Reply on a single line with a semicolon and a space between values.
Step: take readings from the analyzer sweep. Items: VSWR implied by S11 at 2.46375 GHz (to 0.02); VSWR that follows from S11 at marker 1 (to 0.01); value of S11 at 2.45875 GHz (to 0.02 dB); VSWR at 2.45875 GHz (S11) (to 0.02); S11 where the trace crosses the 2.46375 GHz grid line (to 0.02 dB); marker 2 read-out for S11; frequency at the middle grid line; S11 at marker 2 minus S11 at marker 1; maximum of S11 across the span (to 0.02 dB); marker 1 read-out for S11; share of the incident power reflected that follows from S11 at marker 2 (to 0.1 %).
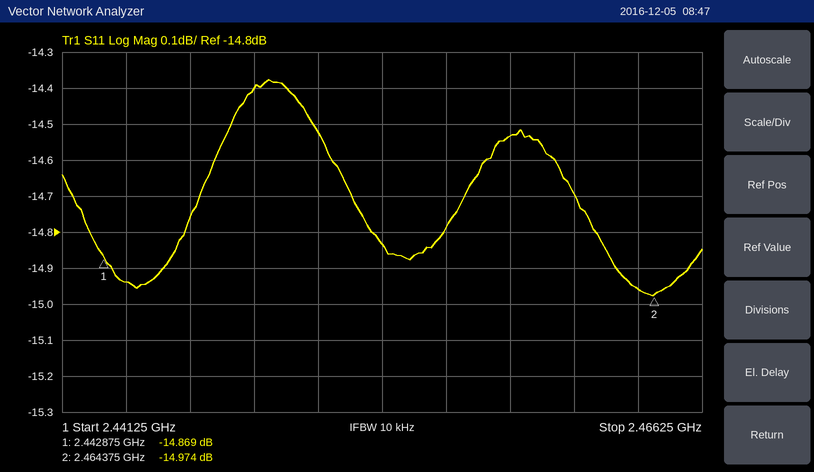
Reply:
1.44; 1.44; -14.54 dB; 1.46; -14.96 dB; -14.974 dB; 2.45375 GHz; -0.105 dB; -14.38 dB; -14.869 dB; 3.2 %
